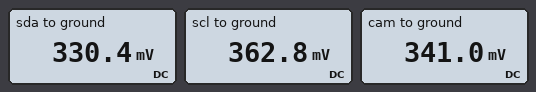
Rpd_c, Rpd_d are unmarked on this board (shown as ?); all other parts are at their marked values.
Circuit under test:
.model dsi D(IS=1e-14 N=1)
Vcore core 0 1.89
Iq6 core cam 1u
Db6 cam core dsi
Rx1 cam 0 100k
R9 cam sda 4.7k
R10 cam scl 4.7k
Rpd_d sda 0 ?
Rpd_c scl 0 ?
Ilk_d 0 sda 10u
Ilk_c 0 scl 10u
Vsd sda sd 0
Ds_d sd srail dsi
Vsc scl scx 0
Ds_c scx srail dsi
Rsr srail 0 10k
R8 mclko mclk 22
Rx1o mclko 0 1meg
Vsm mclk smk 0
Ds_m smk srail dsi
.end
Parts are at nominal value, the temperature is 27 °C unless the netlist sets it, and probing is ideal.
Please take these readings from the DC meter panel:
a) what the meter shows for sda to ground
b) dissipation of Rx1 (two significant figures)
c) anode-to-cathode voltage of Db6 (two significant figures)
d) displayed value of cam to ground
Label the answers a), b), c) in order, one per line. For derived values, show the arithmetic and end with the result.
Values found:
a) 330.4 mV
b) (341 mV)^2 / 100 kΩ = 1.2 µW
c) 341 mV - 1.89 V = -1.5 V
d) 341.0 mV
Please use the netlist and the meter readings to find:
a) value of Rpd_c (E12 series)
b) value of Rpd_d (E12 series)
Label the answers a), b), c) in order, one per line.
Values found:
a) 68 kΩ
b) 27 kΩ
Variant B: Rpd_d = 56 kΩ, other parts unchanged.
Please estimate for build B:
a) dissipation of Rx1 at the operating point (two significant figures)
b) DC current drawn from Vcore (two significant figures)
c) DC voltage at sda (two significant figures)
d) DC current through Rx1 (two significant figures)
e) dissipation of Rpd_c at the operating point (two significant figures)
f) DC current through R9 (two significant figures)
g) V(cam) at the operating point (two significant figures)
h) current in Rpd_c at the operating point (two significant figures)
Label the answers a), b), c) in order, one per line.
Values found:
a) 2.1 µW
b) 1.0 µA
c) 470 mV
d) 4.6 µA
e) 3.3 µW
f) 1.2 µA
g) 460 mV
h) 7.0 µA
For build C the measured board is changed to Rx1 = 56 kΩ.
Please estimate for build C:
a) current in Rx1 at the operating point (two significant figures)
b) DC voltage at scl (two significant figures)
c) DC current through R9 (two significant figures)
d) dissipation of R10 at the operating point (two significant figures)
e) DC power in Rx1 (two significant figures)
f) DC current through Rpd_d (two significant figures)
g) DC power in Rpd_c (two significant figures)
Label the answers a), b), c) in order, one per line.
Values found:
a) 5.3 µA
b) 320 mV
c) 910 nA
d) 130 nW
e) 1.6 µW
f) 11 µA
g) 1.5 µW
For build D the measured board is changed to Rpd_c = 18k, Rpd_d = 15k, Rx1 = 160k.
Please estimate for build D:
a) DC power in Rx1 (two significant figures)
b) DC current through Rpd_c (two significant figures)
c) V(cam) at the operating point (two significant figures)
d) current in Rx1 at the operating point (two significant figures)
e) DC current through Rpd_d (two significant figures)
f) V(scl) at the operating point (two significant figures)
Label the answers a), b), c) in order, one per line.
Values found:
a) 170 nW
b) 9.3 µA
c) 160 mV
d) 1.0 µA
e) 11 µA
f) 170 mV
